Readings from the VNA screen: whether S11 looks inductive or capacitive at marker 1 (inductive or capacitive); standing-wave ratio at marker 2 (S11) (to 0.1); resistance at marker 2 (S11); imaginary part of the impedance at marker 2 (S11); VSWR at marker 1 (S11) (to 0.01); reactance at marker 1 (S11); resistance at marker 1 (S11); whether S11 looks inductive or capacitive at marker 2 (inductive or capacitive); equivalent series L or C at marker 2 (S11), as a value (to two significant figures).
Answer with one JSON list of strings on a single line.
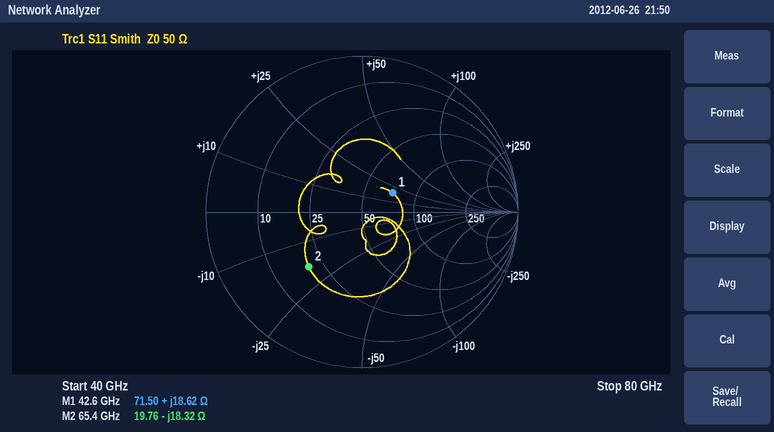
["inductive", "2.9", "19.76 Ω", "-18.32 Ω", "1.60", "+18.62 Ω", "71.50 Ω", "capacitive", "130 fF"]
